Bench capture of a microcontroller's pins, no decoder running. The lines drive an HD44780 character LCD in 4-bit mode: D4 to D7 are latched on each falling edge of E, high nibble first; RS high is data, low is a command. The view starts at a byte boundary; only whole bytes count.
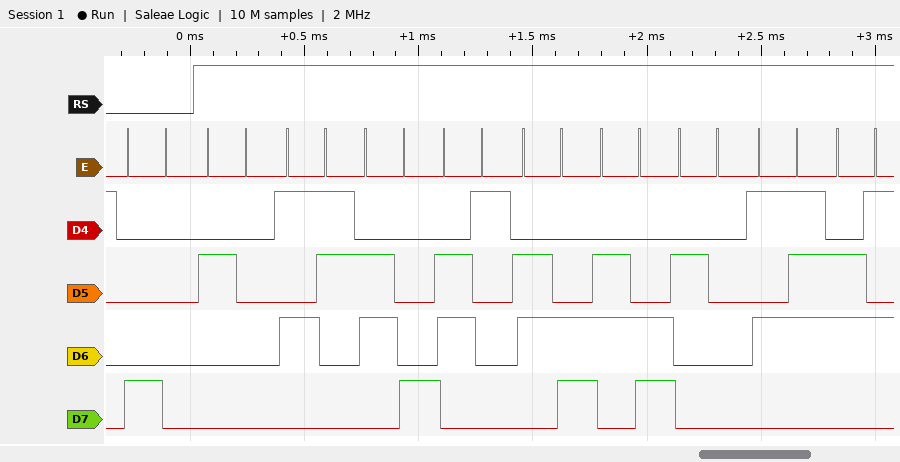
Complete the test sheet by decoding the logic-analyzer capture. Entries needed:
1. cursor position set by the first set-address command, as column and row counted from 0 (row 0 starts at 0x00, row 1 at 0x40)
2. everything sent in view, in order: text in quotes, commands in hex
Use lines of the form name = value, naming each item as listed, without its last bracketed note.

cursor position set by the first set-address command, as column and row counted from 0 = column 0, row 0
everything sent in view, in order: text in quotes, commands in hex = 0x80 " Shall We"
